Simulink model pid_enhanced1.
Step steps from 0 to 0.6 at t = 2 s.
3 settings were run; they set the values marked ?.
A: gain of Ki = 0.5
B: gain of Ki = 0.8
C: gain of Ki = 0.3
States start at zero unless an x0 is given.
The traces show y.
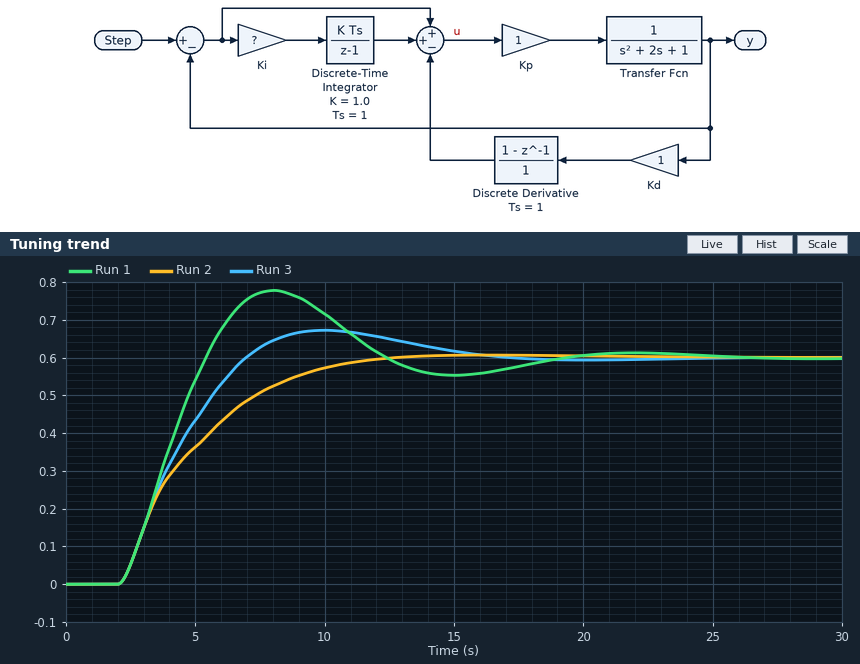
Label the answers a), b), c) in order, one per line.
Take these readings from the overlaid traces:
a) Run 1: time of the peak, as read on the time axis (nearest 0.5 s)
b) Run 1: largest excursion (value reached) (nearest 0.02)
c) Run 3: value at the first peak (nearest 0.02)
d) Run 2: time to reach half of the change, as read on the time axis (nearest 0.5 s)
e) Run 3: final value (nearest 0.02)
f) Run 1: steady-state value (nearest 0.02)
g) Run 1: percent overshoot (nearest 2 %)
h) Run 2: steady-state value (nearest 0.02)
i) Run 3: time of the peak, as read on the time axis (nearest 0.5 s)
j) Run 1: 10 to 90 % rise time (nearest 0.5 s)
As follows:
a) 8.0 s
b) 0.78
c) 0.68
d) 4.0 s
e) 0.60
f) 0.60
g) 30 %
h) 0.60
i) 10.0 s
j) 2.5 s
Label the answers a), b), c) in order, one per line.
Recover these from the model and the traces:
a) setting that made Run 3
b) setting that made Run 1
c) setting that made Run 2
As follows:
a) A
b) B
c) C
